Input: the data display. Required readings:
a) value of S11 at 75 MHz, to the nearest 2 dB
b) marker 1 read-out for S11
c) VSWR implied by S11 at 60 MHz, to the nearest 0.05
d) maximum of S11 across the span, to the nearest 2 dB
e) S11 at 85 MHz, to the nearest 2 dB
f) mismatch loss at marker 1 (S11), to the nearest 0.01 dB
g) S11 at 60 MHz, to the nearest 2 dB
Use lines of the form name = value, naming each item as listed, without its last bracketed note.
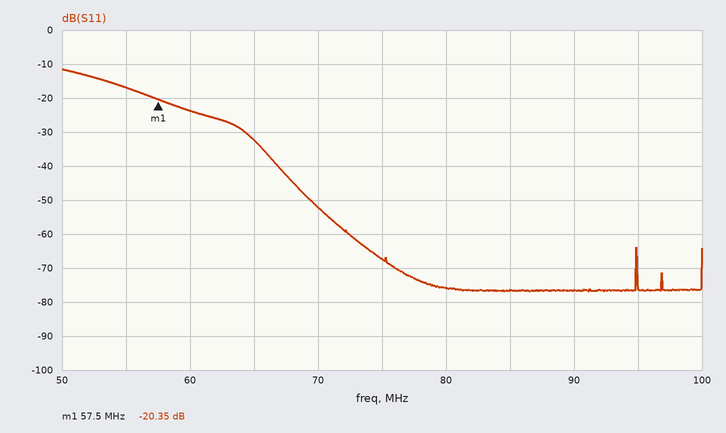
value of S11 at 75 MHz, to the nearest 2 dB = -68 dB
marker 1 read-out for S11 = -20.35 dB
VSWR implied by S11 at 60 MHz, to the nearest 0.05 = 1.15
maximum of S11 across the span, to the nearest 2 dB = -12 dB
S11 at 85 MHz, to the nearest 2 dB = -76 dB
mismatch loss at marker 1 (S11), to the nearest 0.01 dB = 0.04 dB
S11 at 60 MHz, to the nearest 2 dB = -24 dB
